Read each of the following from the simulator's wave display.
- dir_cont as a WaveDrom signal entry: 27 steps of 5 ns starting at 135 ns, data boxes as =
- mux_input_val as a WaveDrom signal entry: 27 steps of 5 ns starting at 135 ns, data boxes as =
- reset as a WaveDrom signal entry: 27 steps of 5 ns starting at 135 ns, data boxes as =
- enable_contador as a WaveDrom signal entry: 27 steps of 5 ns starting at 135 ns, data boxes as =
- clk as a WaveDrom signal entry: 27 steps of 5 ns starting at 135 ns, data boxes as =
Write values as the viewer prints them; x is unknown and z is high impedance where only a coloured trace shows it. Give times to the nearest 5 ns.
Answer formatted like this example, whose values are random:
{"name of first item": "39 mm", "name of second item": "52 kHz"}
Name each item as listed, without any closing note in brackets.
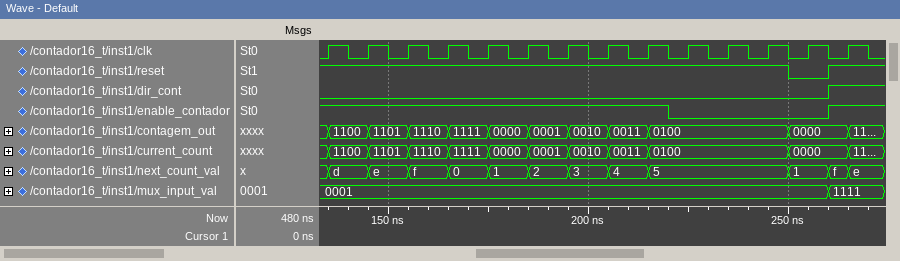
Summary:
{"dir_cont as a WaveDrom signal entry: 27 steps of 5 ns starting at 135 ns, data boxes as =": "{name: 'dir_cont', wave: '0........................1.'}", "mux_input_val as a WaveDrom signal entry: 27 steps of 5 ns starting at 135 ns, data boxes as =": "{name: 'mux_input_val', wave: '=........................=.', data: '0001 1111'}", "reset as a WaveDrom signal entry: 27 steps of 5 ns starting at 135 ns, data boxes as =": "{name: 'reset', wave: '1......................0.1.'}", "enable_contador as a WaveDrom signal entry: 27 steps of 5 ns starting at 135 ns, data boxes as =": "{name: 'enable_contador', wave: '1................0.......1.'}", "clk as a WaveDrom signal entry: 27 steps of 5 ns starting at 135 ns, data boxes as =": "{name: 'clk', wave: '101010101010101010101010101'}"}
